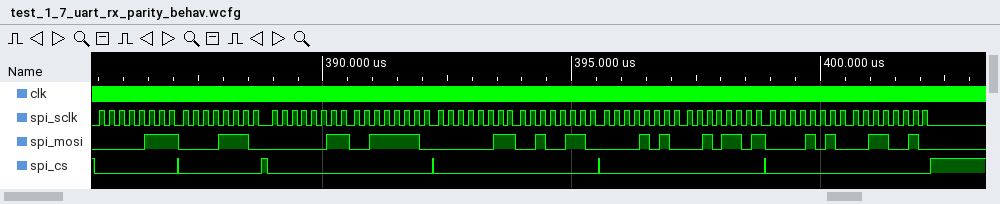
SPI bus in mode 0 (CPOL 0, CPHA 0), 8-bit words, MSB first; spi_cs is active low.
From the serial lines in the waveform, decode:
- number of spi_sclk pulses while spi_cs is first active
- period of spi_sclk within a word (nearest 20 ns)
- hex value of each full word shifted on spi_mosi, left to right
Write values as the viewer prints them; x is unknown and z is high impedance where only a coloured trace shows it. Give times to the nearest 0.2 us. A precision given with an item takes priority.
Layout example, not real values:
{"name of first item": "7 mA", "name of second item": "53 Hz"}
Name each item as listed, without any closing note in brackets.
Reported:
{"number of spi_sclk pulses while spi_cs is first active": "8", "period of spi_sclk within a word": "200 ns", "hex value of each full word shifted on spi_mosi, left to right": "07, 0E, 03, 3E, 03, 26, 0A, 2D, 0A, 32"}
